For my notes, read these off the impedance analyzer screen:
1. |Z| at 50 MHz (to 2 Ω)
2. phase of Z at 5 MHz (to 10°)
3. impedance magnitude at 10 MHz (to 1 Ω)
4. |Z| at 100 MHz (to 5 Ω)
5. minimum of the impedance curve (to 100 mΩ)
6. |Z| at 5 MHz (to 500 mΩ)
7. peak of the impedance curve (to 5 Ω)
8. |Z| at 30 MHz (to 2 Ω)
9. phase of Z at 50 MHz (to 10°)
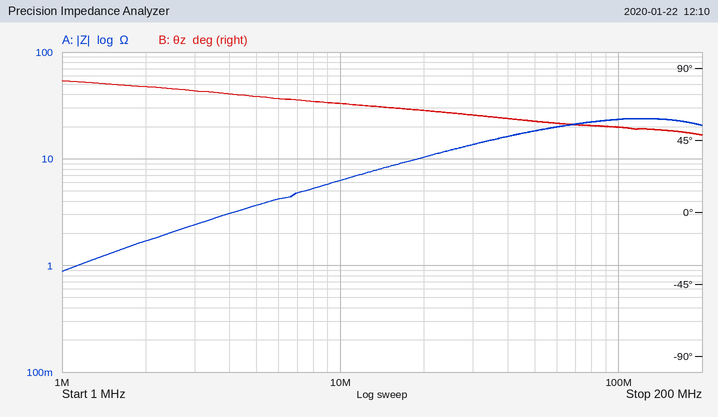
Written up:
18 Ω
70°
6 Ω
25 Ω
900 mΩ
3.5 Ω
25 Ω
14 Ω
60°
